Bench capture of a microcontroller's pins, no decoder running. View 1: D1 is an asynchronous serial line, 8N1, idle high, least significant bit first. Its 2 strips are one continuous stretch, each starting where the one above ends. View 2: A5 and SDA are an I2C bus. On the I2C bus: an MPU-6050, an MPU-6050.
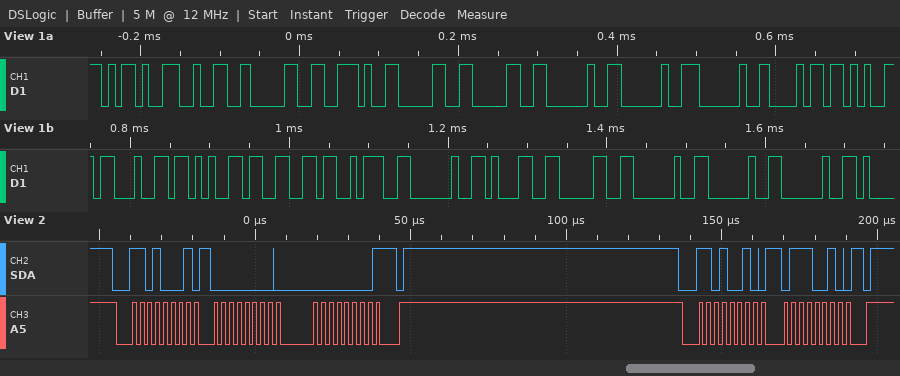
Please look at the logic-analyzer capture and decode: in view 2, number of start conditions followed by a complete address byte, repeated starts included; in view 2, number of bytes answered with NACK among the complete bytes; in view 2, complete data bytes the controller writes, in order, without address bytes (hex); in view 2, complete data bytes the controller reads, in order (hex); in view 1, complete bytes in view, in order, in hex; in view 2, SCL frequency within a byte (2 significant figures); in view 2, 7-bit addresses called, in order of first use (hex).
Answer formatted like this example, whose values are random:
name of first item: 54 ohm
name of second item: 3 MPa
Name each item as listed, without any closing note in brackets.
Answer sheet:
in view 2, number of start conditions followed by a complete address byte, repeated starts included: 2
in view 2, number of bytes answered with NACK among the complete bytes: 1
in view 2, complete data bytes the controller writes, in order, without address bytes: 72
in view 2, complete data bytes the controller reads, in order: 00 00
in view 1, complete bytes in view, in order, in hex: 2D 32 30 2E 30 30 20 20 20 68 65 64 65 66 3A 20 31 30 20 20 20
in view 2, SCL frequency within a byte: 400 kHz
in view 2, 7-bit addresses called, in order of first use: 0x68 0x69
